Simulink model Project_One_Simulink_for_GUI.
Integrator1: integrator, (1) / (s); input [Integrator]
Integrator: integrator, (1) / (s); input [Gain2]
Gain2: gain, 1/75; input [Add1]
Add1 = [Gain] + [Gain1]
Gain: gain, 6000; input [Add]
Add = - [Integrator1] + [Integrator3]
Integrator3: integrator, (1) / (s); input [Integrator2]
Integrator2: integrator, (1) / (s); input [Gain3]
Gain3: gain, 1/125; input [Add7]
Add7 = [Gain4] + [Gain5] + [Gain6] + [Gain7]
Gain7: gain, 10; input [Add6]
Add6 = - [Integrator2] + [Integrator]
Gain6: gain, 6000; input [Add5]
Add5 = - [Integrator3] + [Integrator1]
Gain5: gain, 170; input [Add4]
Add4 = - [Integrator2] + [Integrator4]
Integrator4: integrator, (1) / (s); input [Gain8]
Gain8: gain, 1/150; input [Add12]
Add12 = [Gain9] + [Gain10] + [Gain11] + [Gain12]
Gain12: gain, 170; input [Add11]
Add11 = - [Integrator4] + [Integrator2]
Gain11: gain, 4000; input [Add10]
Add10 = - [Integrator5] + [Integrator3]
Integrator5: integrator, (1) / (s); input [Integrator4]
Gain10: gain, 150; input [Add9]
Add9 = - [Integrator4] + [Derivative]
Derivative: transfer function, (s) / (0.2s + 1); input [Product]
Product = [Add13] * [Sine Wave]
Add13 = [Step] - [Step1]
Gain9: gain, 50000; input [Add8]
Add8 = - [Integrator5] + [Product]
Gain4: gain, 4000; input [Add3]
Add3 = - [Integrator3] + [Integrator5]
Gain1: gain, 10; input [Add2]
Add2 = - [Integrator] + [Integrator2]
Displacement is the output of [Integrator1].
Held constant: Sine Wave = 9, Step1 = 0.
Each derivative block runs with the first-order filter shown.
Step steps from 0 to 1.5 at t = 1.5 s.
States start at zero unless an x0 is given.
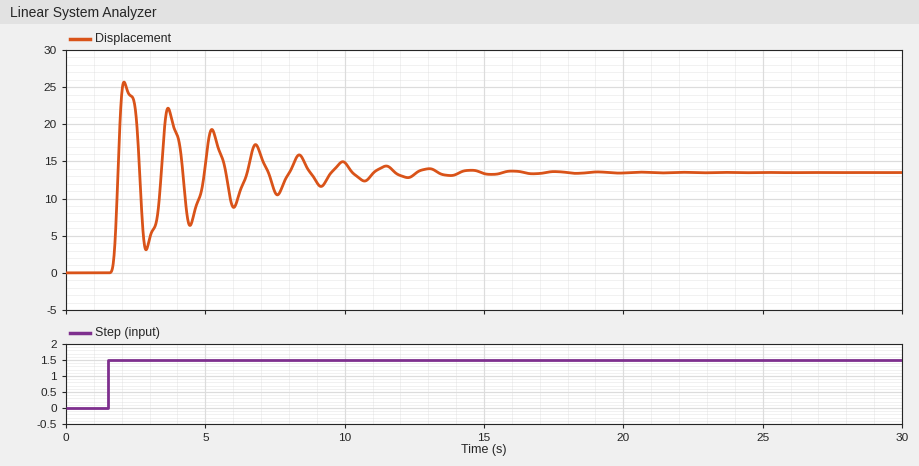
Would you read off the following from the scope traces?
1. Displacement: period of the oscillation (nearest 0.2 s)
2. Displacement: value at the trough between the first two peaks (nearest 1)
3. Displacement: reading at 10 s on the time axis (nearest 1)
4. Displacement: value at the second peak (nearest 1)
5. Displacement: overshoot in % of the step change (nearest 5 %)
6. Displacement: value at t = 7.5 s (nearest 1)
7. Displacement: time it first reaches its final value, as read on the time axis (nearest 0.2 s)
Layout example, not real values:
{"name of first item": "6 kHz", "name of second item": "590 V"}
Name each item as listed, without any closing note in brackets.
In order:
{"Displacement: period of the oscillation": "1.6 s", "Displacement: value at the trough between the first two peaks": "3", "Displacement: reading at 10 s on the time axis": "15", "Displacement: value at the second peak": "22", "Displacement: overshoot in % of the step change": "90 %", "Displacement: value at t = 7.5 s": "11", "Displacement: time it first reaches its final value, as read on the time axis": "1.8 s"}
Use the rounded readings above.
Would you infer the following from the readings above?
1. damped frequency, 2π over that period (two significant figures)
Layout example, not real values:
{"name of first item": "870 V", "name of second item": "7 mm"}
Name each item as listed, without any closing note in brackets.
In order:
{"damped frequency, 2π over that period": "3.9 rad/s"}
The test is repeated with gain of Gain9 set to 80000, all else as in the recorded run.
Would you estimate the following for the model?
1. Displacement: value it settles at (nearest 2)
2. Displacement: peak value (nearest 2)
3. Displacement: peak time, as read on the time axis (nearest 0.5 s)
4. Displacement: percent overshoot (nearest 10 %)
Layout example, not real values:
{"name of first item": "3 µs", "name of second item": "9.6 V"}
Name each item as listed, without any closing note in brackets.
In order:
{"Displacement: value it settles at": "14", "Displacement: peak value": "26", "Displacement: peak time, as read on the time axis": "2.0 s", "Displacement: percent overshoot": "90 %"}
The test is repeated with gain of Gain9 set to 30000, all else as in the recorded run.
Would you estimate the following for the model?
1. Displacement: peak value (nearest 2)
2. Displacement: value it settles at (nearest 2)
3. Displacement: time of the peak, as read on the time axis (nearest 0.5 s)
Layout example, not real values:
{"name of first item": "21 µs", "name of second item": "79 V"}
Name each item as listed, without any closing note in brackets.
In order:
{"Displacement: peak value": "28", "Displacement: value it settles at": "14", "Displacement: time of the peak, as read on the time axis": "2.0 s"}
